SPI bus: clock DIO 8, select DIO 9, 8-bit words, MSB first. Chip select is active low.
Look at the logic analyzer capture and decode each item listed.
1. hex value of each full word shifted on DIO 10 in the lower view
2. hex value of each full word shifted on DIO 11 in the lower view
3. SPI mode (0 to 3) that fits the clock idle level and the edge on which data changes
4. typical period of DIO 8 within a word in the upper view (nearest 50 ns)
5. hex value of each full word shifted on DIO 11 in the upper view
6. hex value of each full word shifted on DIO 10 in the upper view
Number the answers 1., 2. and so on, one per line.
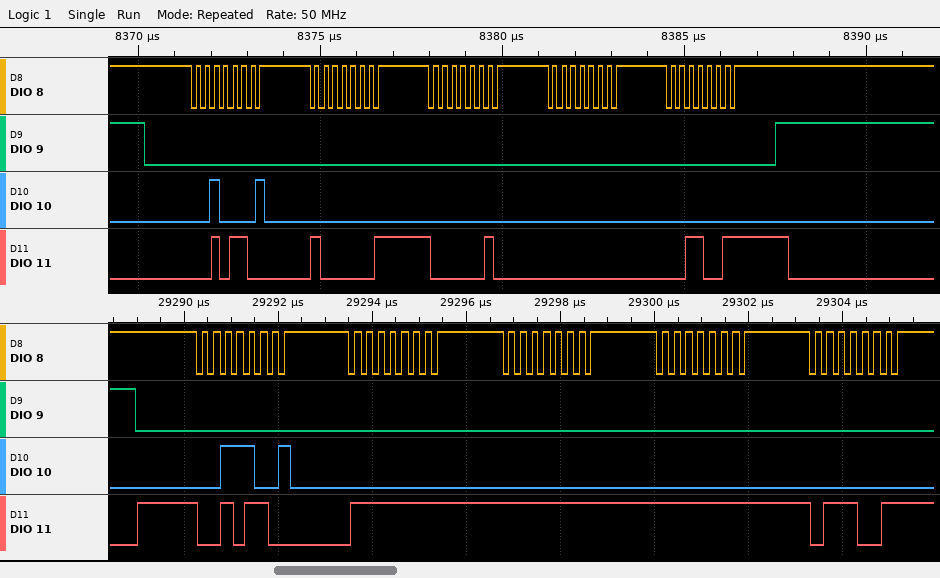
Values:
1. 39, 00, 00, 00, 00
2. 2C, FF, FF, FF, 73
3. 3
4. 250 ns
5. 2C, 81, 02, 00, 33
6. 21, 00, 00, 00, 00
